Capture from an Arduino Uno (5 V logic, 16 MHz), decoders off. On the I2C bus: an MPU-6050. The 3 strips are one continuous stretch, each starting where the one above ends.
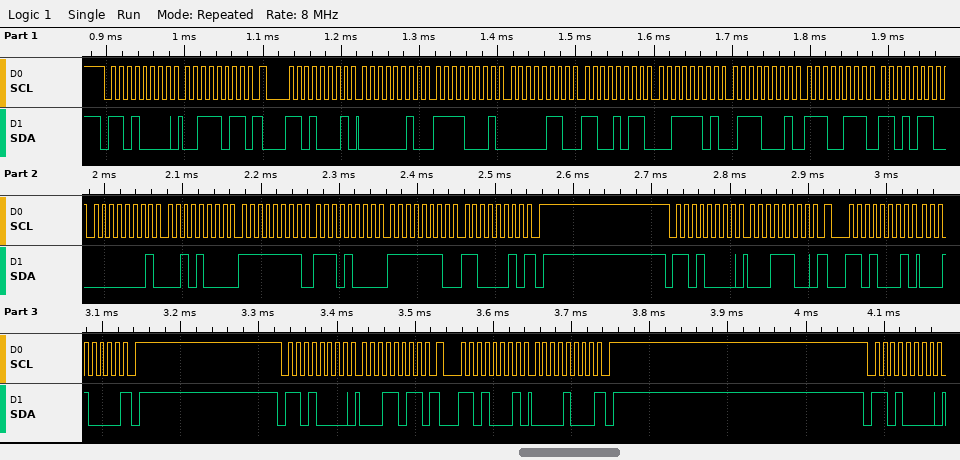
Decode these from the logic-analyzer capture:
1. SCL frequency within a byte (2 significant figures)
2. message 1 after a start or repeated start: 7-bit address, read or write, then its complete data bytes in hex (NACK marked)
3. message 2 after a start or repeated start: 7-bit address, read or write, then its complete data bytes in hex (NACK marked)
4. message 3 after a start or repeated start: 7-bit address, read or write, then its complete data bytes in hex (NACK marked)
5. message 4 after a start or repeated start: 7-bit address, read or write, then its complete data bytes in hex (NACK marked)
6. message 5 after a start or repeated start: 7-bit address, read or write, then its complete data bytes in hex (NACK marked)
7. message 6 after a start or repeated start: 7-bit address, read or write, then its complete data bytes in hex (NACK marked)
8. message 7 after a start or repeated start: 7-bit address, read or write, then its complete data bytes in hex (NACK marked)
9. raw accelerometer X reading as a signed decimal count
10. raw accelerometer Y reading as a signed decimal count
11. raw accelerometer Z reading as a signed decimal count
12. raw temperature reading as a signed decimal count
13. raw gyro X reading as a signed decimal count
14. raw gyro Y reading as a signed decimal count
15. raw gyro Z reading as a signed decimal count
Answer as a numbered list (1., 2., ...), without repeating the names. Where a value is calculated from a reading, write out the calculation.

1. 100 kHz
2. 0x68 write: 3B
3. 0x68 read: 02 F1 06 CB 3D 71 E7 D6 01 28 FF E8 FE C2 NACK
4. 0x68 write: 1C
5. 0x68 read: 10 NACK
6. 0x68 write: 1B
7. 0x68 read: 08 NACK
8. 0x68 write
9. 0x02F1 = 753
10. 0x06CB = 1739
11. 0x3D71 = 15729
12. 0xE7D6 = -6186
13. 0x0128 = 296
14. 0xFFE8 = -24
15. 0xFEC2 = -318
